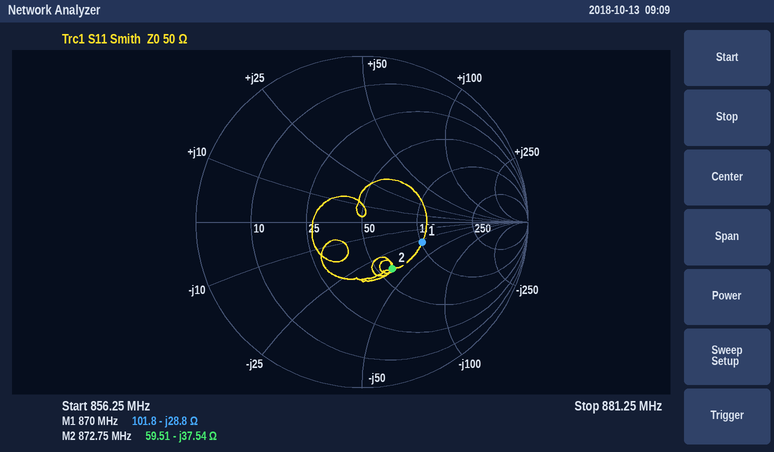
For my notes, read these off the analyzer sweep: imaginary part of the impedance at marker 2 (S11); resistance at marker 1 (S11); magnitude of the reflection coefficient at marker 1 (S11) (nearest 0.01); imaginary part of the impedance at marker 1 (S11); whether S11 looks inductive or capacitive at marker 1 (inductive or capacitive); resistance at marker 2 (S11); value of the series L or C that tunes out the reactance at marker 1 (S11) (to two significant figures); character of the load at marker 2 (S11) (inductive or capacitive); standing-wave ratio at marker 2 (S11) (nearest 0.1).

-37.54 Ω
101.8 Ω
0.38
-28.8 Ω
capacitive
59.51 Ω
5.3 nH
capacitive
2.0
